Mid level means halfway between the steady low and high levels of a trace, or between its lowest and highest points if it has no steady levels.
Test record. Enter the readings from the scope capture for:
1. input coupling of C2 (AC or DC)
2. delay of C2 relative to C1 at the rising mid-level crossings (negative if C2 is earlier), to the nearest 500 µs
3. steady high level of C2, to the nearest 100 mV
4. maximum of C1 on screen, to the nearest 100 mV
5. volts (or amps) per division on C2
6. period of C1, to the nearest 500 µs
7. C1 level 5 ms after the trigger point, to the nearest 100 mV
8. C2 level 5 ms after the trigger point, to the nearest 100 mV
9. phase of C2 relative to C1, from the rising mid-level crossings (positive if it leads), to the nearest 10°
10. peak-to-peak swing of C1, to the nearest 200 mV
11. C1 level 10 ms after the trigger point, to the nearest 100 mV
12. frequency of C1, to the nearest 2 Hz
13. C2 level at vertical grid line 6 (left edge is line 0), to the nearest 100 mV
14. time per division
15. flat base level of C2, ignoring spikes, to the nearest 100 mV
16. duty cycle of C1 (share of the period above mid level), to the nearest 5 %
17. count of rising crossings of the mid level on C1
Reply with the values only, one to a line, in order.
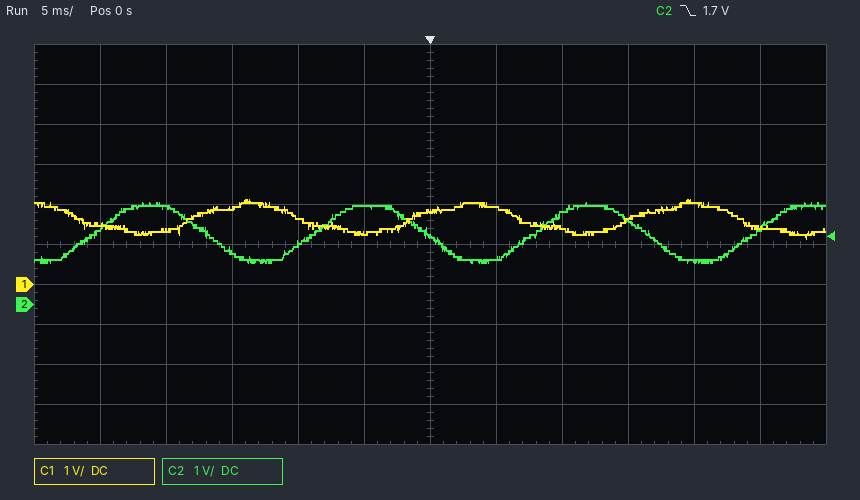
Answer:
DC
-7.0 ms
2.5 V
2.1 V
1 V
16.5 ms
1.9 V
1.2 V
+150°
1.0 V
1.4 V
60 Hz
1.7 V
5 ms
1.1 V
50 %
3
